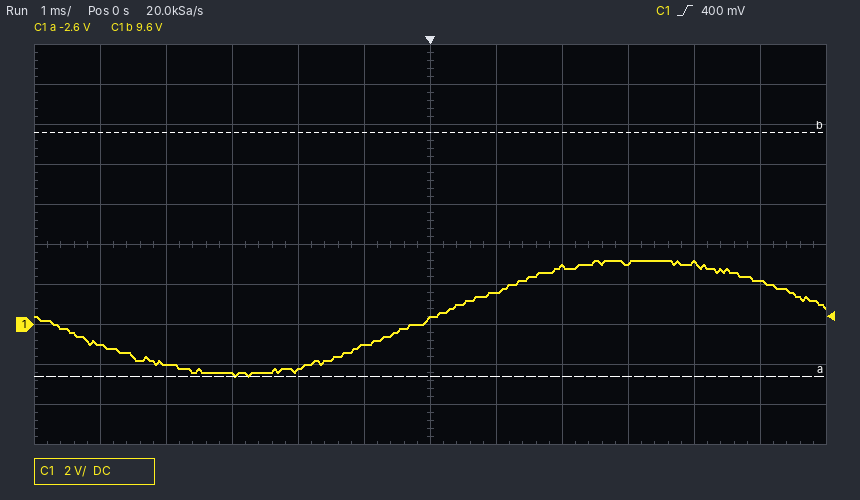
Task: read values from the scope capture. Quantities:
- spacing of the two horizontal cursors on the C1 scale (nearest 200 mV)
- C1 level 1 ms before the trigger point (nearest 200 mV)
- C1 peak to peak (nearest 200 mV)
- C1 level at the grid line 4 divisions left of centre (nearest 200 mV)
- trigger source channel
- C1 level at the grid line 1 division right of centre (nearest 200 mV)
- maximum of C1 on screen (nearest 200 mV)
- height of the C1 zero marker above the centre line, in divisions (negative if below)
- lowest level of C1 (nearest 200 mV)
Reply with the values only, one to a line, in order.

12.2 V
-1.0 V
5.8 V
-2.0 V
C1
1.6 V
3.2 V
-2.0 div
-2.6 V
